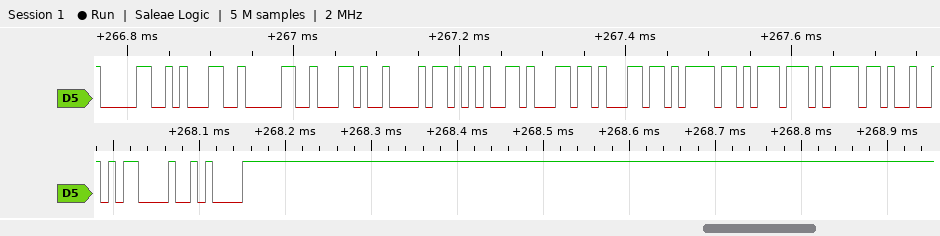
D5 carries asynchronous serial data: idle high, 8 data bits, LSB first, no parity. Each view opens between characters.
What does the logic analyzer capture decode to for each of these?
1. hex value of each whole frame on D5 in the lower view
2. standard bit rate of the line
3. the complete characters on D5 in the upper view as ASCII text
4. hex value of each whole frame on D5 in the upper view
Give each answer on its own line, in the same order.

0D, 0A
115200 baud
"010,hellowo"
30, 31, 30, 2C, 68, 65, 6C, 6C, 6F, 77, 6F
